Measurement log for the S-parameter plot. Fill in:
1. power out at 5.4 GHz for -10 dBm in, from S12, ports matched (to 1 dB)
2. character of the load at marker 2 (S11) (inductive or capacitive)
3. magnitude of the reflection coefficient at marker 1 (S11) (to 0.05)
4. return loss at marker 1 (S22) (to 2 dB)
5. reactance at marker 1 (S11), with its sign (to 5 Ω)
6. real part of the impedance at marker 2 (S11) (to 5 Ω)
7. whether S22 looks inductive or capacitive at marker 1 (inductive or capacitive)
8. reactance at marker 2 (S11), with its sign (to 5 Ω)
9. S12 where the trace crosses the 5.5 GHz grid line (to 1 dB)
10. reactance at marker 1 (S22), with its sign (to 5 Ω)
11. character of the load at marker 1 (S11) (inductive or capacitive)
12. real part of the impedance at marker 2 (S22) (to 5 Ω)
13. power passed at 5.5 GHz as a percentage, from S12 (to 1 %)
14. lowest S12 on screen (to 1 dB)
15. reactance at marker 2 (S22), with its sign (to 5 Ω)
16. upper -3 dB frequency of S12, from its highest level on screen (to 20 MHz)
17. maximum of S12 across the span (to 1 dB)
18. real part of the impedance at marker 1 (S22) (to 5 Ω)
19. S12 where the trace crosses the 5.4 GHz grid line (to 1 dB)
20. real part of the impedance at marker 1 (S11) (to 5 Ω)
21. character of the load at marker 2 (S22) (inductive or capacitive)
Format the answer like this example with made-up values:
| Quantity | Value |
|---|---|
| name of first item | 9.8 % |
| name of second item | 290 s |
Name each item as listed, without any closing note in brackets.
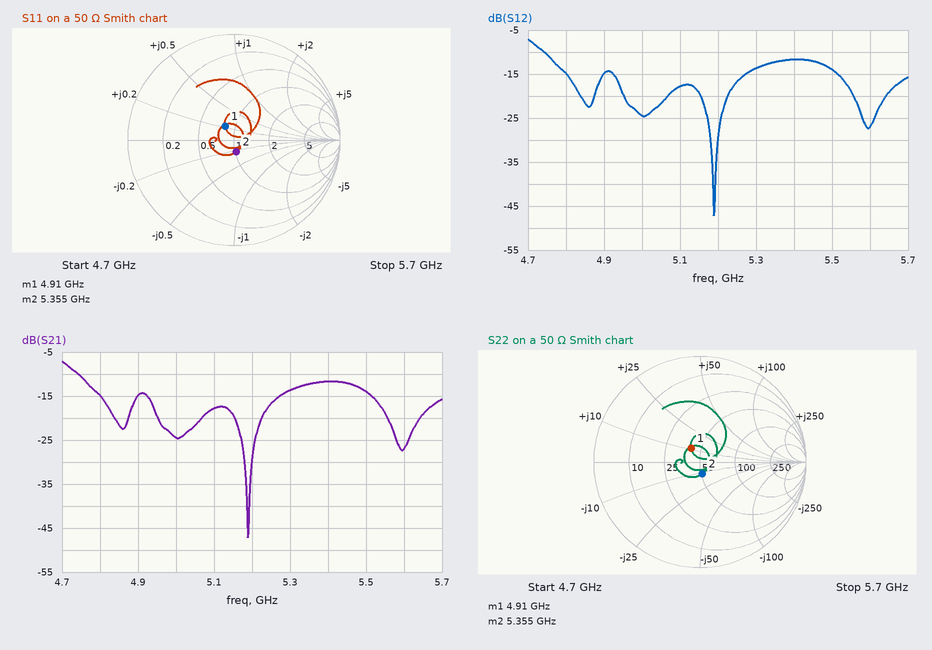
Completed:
| Quantity | Value |
|---|---|
| power out at 5.4 GHz for -10 dBm in, from S12, ports matched | -22 dBm |
| character of the load at marker 2 (S11) | capacitive |
| magnitude of the reflection coefficient at marker 1 (S11) | 0.15 |
| return loss at marker 1 (S22) | 16 dB |
| reactance at marker 1 (S11), with its sign | +10 Ω |
| real part of the impedance at marker 2 (S11) | 50 Ω |
| whether S22 looks inductive or capacitive at marker 1 | inductive |
| reactance at marker 2 (S11), with its sign | -10 Ω |
| S12 where the trace crosses the 5.5 GHz grid line | -14 dB |
| reactance at marker 1 (S22), with its sign | +10 Ω |
| character of the load at marker 1 (S11) | inductive |
| real part of the impedance at marker 2 (S22) | 50 Ω |
| power passed at 5.5 GHz as a percentage, from S12 | 4 % |
| lowest S12 on screen | -47 dB |
| reactance at marker 2 (S22), with its sign | -10 Ω |
| upper -3 dB frequency of S12, from its highest level on screen | 4.74 GHz |
| maximum of S12 across the span | -7 dB |
| real part of the impedance at marker 1 (S22) | 40 Ω |
| S12 where the trace crosses the 5.4 GHz grid line | -12 dB |
| real part of the impedance at marker 1 (S11) | 40 Ω |
| character of the load at marker 2 (S22) | capacitive |
